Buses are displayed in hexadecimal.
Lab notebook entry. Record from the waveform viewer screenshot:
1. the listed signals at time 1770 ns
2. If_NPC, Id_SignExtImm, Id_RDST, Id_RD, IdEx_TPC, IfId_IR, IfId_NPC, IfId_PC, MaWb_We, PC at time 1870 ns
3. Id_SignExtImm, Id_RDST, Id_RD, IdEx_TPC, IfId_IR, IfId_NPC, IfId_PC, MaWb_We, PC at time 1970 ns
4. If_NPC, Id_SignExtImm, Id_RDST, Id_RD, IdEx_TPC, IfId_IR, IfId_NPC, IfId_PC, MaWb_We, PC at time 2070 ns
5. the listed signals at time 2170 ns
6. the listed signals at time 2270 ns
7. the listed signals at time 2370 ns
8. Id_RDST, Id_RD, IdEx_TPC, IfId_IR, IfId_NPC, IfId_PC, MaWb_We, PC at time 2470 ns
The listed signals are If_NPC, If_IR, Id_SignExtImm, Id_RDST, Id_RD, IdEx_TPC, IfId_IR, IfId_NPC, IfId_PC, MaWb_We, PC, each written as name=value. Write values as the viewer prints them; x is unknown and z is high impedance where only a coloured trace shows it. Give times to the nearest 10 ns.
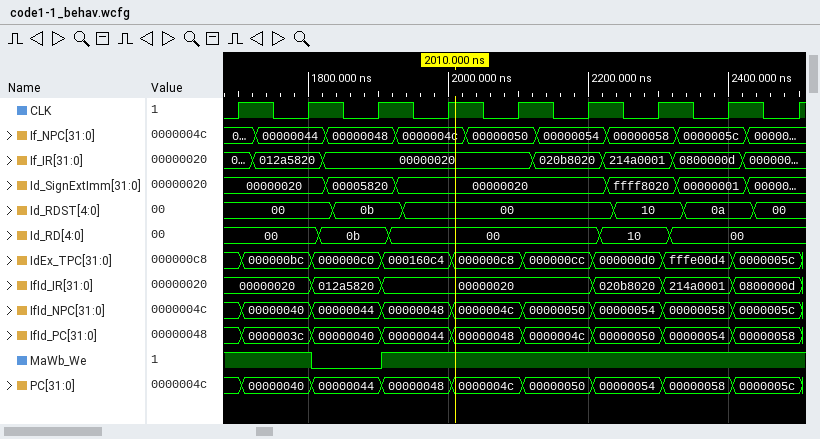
If_NPC=00000044, If_IR=012a5820, Id_SignExtImm=00000020, Id_RDST=00, Id_RD=00, IdEx_TPC=000000bc, IfId_IR=00000020, IfId_NPC=00000040, IfId_PC=0000003c, MaWb_We=1, PC=00000040
If_NPC=00000048, Id_SignExtImm=00005820, Id_RDST=0b, Id_RD=0b, IdEx_TPC=000000c0, IfId_IR=012a5820, IfId_NPC=00000044, IfId_PC=00000040, MaWb_We=0, PC=00000044
Id_SignExtImm=00000020, Id_RDST=00, Id_RD=00, IdEx_TPC=000160c4, IfId_IR=00000020, IfId_NPC=00000048, IfId_PC=00000044, MaWb_We=1, PC=00000048
If_NPC=00000050, Id_SignExtImm=00000020, Id_RDST=00, Id_RD=00, IdEx_TPC=000000c8, IfId_IR=00000020, IfId_NPC=0000004c, IfId_PC=00000048, MaWb_We=1, PC=0000004c
If_NPC=00000054, If_IR=020b8020, Id_SignExtImm=00000020, Id_RDST=00, Id_RD=00, IdEx_TPC=000000cc, IfId_IR=00000020, IfId_NPC=00000050, IfId_PC=0000004c, MaWb_We=1, PC=00000050
If_NPC=00000058, If_IR=214a0001, Id_SignExtImm=ffff8020, Id_RDST=10, Id_RD=10, IdEx_TPC=000000d0, IfId_IR=020b8020, IfId_NPC=00000054, IfId_PC=00000050, MaWb_We=1, PC=00000054
If_NPC=0000005c, If_IR=0800000d, Id_SignExtImm=00000001, Id_RDST=0a, Id_RD=00, IdEx_TPC=fffe00d4, IfId_IR=214a0001, IfId_NPC=00000058, IfId_PC=00000054, MaWb_We=1, PC=00000058
Id_RDST=00, Id_RD=00, IdEx_TPC=0000005c, IfId_IR=0800000d, IfId_NPC=0000005c, IfId_PC=00000058, MaWb_We=1, PC=0000005c
